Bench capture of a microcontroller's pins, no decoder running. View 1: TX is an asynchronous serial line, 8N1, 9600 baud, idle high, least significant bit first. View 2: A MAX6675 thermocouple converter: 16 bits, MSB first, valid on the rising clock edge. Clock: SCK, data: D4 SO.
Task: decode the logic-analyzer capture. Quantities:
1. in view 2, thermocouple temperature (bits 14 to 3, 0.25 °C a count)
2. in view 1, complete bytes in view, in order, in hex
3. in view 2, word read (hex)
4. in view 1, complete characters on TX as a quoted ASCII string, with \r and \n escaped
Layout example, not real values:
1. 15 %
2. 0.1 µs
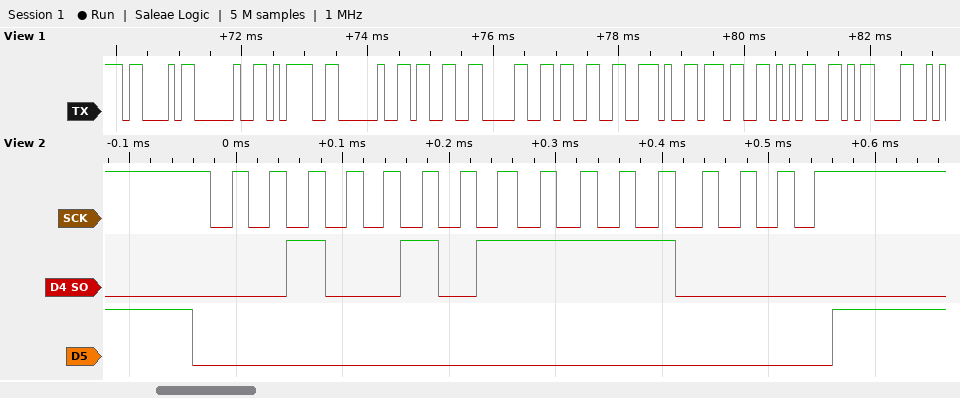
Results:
1. 303.50 °C
2. 43 20 3D 20 33 30 33 2E 37 35 0D
3. 0x25F0
4. "C = 303.75\r"
